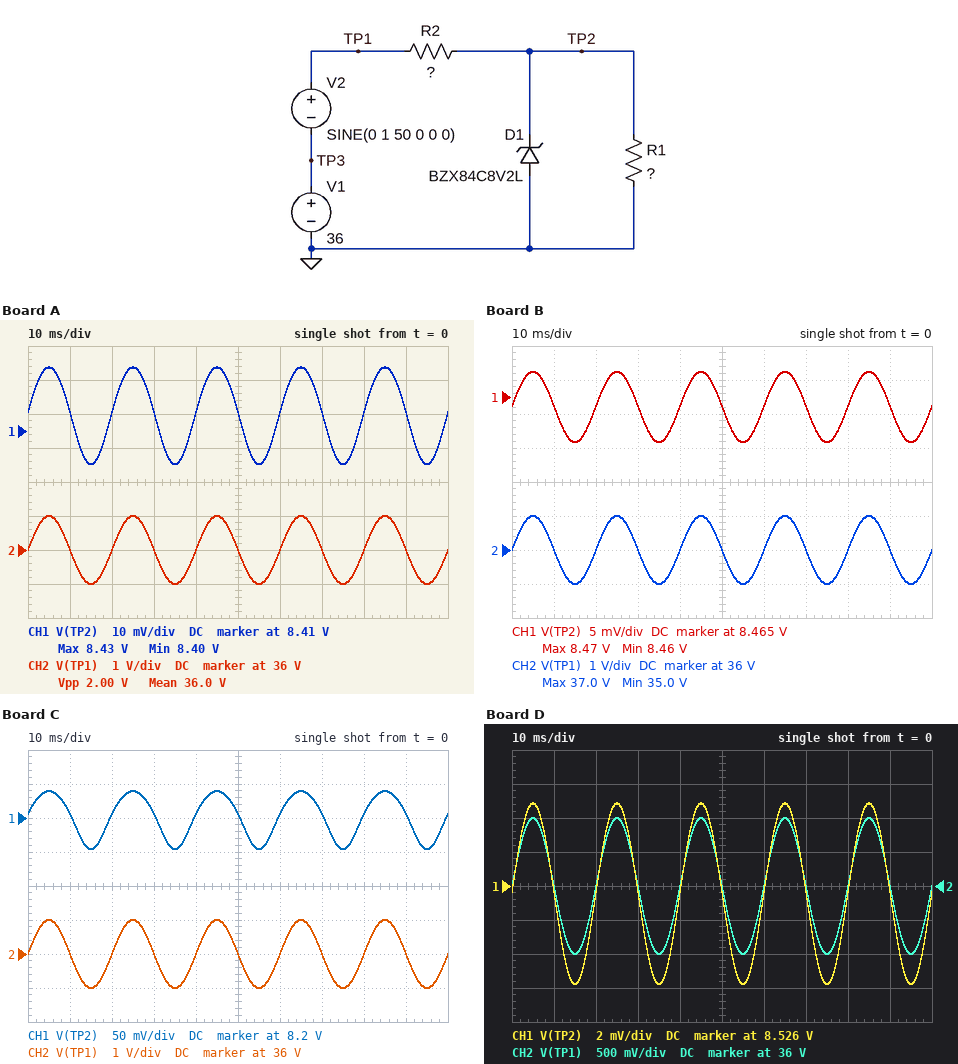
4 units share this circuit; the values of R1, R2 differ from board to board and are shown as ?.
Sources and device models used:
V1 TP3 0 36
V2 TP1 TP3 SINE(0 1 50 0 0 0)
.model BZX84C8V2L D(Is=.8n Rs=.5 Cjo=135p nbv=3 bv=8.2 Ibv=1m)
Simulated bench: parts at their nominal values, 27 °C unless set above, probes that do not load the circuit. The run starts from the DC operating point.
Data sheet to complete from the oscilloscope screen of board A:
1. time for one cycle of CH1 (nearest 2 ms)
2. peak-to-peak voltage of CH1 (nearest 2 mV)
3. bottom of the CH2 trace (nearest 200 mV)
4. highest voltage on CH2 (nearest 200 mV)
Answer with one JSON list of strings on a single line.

["20 ms", "28 mV", "35.0 V", "37.0 V"]
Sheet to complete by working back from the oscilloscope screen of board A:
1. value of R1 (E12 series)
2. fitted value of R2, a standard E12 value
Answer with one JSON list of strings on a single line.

["150 Ω", "390 Ω"]
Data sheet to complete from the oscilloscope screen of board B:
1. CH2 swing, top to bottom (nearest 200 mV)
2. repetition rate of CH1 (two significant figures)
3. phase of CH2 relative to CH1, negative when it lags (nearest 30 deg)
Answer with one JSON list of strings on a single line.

["2.0 V", "50 Hz", "0 deg"]
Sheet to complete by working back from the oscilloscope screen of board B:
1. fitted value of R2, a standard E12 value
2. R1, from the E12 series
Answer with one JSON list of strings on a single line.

["680 Ω", "560 Ω"]
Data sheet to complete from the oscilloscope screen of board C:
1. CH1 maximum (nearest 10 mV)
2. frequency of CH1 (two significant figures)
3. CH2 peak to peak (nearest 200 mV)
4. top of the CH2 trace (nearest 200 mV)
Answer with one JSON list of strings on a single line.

["8.24 V", "50 Hz", "2.0 V", "37.0 V"]
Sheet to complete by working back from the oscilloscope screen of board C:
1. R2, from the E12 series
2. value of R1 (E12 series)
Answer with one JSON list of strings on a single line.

["1.5 kΩ", "470 Ω"]
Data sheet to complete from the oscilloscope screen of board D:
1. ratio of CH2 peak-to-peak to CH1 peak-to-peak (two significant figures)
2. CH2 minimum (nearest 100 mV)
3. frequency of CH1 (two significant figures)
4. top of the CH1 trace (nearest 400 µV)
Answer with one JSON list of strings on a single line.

["190", "35.0 V", "50 Hz", "8.5308 V"]
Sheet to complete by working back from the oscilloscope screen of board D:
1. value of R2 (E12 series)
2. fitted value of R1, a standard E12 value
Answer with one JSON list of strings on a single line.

["390 Ω", "390 Ω"]
